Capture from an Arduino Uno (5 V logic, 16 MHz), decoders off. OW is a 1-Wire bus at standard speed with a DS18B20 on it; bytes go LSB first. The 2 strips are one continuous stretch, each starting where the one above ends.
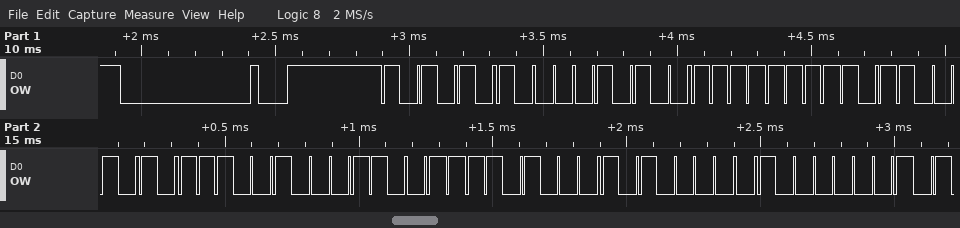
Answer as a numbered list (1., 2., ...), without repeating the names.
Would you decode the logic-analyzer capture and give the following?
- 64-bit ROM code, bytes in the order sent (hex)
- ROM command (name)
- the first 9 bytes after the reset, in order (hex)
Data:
1. 28 FF 4D 9D 98 17 05 81
2. Match ROM
3. 55 28 FF 4D 9D 98 17 05 81
